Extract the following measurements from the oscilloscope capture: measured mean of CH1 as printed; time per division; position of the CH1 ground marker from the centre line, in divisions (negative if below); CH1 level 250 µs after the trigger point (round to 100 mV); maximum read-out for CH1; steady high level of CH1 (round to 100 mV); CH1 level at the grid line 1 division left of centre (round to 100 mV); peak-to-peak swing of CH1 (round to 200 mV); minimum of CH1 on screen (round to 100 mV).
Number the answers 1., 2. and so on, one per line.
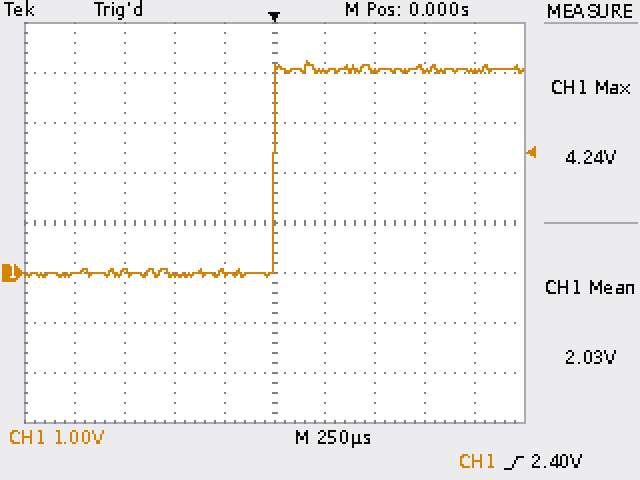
1. 2.03 V
2. 250 µs
3. -1.0 div
4. 4.0 V
5. 4.24 V
6. 4.1 V
7. 0.0 V
8. 4.4 V
9. -100 mV
